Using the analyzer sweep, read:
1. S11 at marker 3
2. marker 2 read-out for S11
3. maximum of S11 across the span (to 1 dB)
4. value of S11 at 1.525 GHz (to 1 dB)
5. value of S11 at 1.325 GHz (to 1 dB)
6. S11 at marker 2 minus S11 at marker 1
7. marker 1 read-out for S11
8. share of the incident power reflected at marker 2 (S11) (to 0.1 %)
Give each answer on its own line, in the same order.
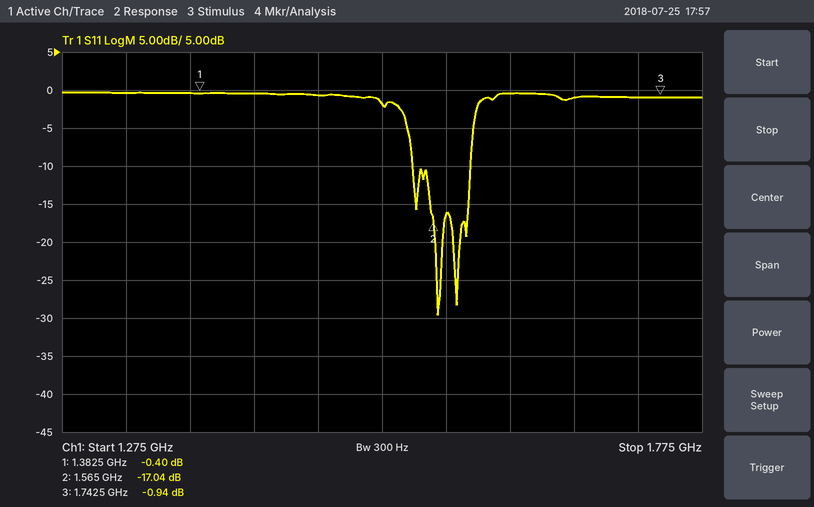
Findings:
-0.94 dB
-17.04 dB
0 dB
-2 dB
0 dB
-16.64 dB
-0.40 dB
2.0 %
